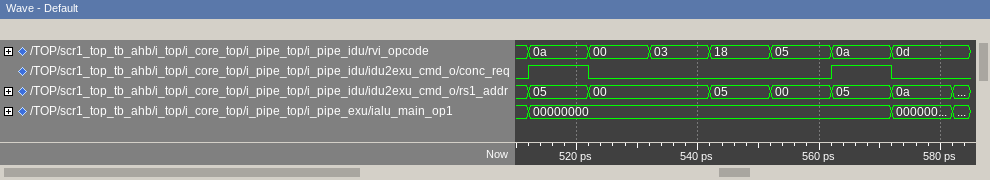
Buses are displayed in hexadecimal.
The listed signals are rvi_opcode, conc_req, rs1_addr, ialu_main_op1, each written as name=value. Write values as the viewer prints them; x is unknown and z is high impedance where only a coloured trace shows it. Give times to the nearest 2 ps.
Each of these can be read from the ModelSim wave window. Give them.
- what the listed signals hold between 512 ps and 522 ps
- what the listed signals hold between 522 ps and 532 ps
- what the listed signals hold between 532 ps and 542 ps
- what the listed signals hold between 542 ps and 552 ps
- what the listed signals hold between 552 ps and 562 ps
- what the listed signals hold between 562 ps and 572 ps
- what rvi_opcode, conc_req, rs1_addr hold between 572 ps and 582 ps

rvi_opcode=0a, conc_req=1, rs1_addr=05, ialu_main_op1=00000000
rvi_opcode=00, conc_req=0, rs1_addr=00, ialu_main_op1=00000000
rvi_opcode=03, conc_req=0, rs1_addr=00, ialu_main_op1=00000000
rvi_opcode=18, conc_req=0, rs1_addr=05, ialu_main_op1=00000000
rvi_opcode=05, conc_req=0, rs1_addr=00, ialu_main_op1=00000000
rvi_opcode=0a, conc_req=1, rs1_addr=05, ialu_main_op1=00000000
rvi_opcode=0d, conc_req=0, rs1_addr=0a
